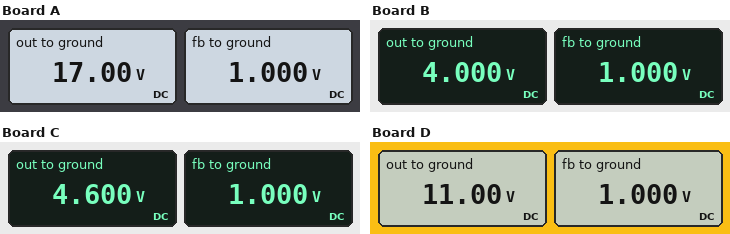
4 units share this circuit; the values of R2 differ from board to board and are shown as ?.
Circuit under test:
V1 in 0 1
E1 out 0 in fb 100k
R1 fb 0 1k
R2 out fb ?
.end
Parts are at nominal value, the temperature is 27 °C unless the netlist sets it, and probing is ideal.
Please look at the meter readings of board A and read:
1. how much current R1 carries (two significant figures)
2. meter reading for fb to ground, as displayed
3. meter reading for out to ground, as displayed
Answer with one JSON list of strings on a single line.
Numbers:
["1.0 mA", "1.000 V", "17.00 V"]
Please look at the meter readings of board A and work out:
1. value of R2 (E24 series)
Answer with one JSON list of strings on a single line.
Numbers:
["16 kΩ"]
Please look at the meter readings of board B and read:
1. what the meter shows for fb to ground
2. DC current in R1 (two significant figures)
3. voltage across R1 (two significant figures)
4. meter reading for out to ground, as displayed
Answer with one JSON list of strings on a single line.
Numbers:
["1.000 V", "1.0 mA", "1.0 V", "4.000 V"]
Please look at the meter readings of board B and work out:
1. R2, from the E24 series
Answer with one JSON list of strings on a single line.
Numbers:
["3 kΩ"]
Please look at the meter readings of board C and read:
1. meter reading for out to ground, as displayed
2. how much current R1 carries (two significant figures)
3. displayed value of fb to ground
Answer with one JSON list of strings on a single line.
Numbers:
["4.600 V", "1.0 mA", "1.000 V"]
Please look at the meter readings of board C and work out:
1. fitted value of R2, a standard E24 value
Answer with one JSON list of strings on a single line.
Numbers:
["3.6 kΩ"]
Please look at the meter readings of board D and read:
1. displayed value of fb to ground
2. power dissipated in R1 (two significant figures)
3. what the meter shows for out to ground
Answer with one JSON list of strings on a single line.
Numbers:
["1.000 V", "1.0 mW", "11.00 V"]
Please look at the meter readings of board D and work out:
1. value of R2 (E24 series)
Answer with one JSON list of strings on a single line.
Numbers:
["10 kΩ"]
